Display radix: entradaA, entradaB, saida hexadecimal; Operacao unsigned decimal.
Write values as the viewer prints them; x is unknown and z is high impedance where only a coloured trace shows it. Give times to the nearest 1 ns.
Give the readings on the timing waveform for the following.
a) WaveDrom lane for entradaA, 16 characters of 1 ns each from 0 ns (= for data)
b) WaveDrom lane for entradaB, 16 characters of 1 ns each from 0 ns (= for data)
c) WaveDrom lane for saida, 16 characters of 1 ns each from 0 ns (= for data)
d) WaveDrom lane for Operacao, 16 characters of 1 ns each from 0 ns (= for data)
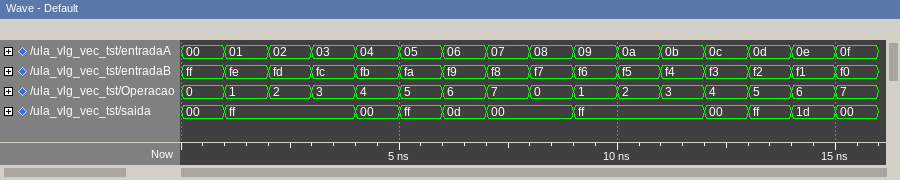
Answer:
{name: 'entradaA', wave: '================', data: '00 01 02 03 04 05 06 07 08 09 0a 0b 0c 0d 0e 0f'}
{name: 'entradaB', wave: '================', data: 'ff fe fd fc fb fa f9 f8 f7 f6 f5 f4 f3 f2 f1 f0'}
{name: 'saida', wave: '==..====.=..====', data: '00 ff 00 ff 0d 00 ff 00 ff 1d 00'}
{name: 'Operacao', wave: '================', data: '0 1 2 3 4 5 6 7 0 1 2 3 4 5 6 7'}
